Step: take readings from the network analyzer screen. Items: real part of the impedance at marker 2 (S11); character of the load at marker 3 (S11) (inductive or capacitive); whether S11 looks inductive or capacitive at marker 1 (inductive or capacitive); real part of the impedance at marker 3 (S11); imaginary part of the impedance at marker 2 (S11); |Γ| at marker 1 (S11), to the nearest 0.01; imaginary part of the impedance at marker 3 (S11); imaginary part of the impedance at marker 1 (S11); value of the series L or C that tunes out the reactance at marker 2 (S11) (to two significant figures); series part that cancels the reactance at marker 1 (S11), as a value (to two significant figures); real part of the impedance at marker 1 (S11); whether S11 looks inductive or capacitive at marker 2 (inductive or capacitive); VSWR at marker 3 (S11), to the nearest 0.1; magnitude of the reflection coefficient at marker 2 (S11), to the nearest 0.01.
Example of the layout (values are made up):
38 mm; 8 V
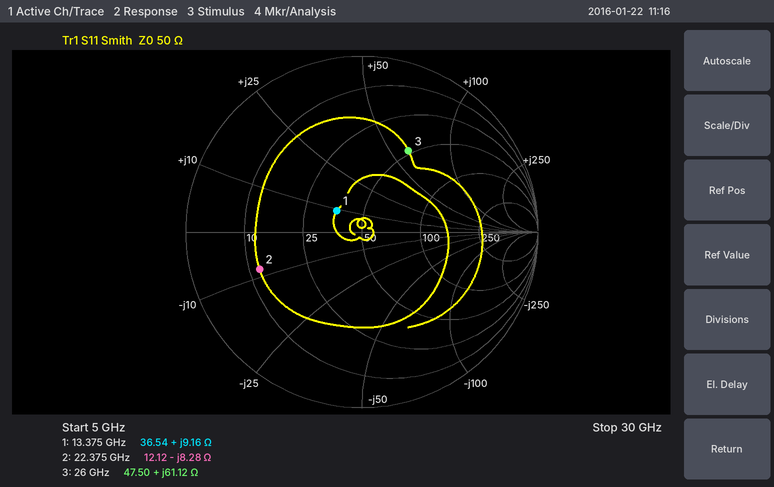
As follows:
12.12 Ω; inductive; inductive; 47.50 Ω; -8.28 Ω; 0.19; +61.12 Ω; +9.16 Ω; 59 pH; 1.3 pF; 36.54 Ω; capacitive; 3.3; 0.62
